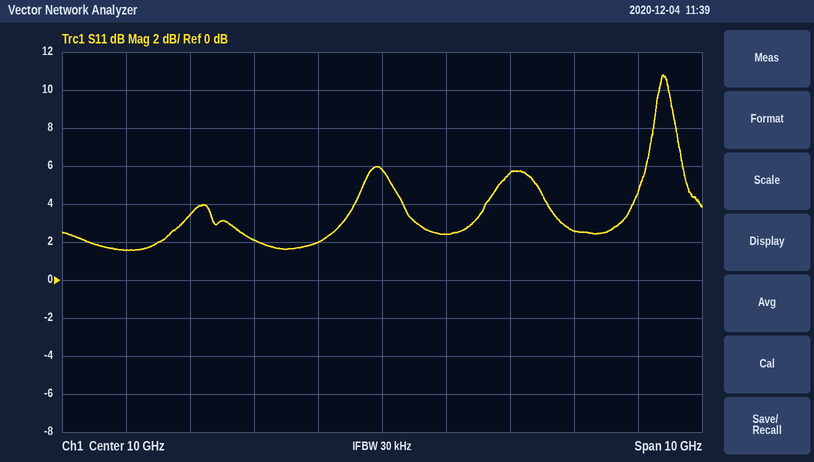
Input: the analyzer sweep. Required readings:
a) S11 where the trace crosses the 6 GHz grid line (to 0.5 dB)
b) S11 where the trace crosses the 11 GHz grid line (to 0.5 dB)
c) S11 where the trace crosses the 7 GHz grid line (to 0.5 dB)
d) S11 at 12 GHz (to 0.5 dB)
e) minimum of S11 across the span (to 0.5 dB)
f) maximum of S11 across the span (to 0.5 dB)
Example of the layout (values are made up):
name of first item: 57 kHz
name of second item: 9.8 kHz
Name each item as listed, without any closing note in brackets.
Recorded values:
S11 where the trace crosses the 6 GHz grid line: 1.5 dB
S11 where the trace crosses the 11 GHz grid line: 2.5 dB
S11 where the trace crosses the 7 GHz grid line: 3.5 dB
S11 at 12 GHz: 5.5 dB
minimum of S11 across the span: 1.5 dB
maximum of S11 across the span: 11.0 dB
